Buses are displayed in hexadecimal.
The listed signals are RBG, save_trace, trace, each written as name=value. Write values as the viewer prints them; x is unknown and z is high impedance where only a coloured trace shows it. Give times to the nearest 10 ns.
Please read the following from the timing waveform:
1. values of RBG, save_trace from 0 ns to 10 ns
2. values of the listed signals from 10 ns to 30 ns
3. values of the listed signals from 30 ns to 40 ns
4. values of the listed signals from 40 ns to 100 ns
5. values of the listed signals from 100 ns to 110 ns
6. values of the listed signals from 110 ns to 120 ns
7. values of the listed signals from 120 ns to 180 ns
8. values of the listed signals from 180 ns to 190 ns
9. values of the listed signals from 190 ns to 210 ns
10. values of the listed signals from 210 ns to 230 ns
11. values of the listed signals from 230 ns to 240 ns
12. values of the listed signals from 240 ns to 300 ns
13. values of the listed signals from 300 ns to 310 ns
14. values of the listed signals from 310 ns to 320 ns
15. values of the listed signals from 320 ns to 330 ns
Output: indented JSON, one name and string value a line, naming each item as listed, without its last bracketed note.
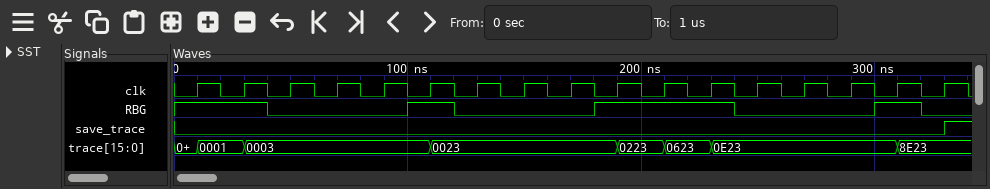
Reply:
{
  "values of RBG, save_trace from 0 ns to 10 ns": "RBG=1, save_trace=0",
  "values of the listed signals from 10 ns to 30 ns": "RBG=1, save_trace=0, trace=0001",
  "values of the listed signals from 30 ns to 40 ns": "RBG=1, save_trace=0, trace=0003",
  "values of the listed signals from 40 ns to 100 ns": "RBG=0, save_trace=0, trace=0003",
  "values of the listed signals from 100 ns to 110 ns": "RBG=1, save_trace=0, trace=0003",
  "values of the listed signals from 110 ns to 120 ns": "RBG=1, save_trace=0, trace=0023",
  "values of the listed signals from 120 ns to 180 ns": "RBG=0, save_trace=0, trace=0023",
  "values of the listed signals from 180 ns to 190 ns": "RBG=1, save_trace=0, trace=0023",
  "values of the listed signals from 190 ns to 210 ns": "RBG=1, save_trace=0, trace=0223",
  "values of the listed signals from 210 ns to 230 ns": "RBG=1, save_trace=0, trace=0623",
  "values of the listed signals from 230 ns to 240 ns": "RBG=1, save_trace=0, trace=0E23",
  "values of the listed signals from 240 ns to 300 ns": "RBG=0, save_trace=0, trace=0E23",
  "values of the listed signals from 300 ns to 310 ns": "RBG=1, save_trace=0, trace=0E23",
  "values of the listed signals from 310 ns to 320 ns": "RBG=1, save_trace=0, trace=8E23",
  "values of the listed signals from 320 ns to 330 ns": "RBG=0, save_trace=0, trace=8E23"
}
